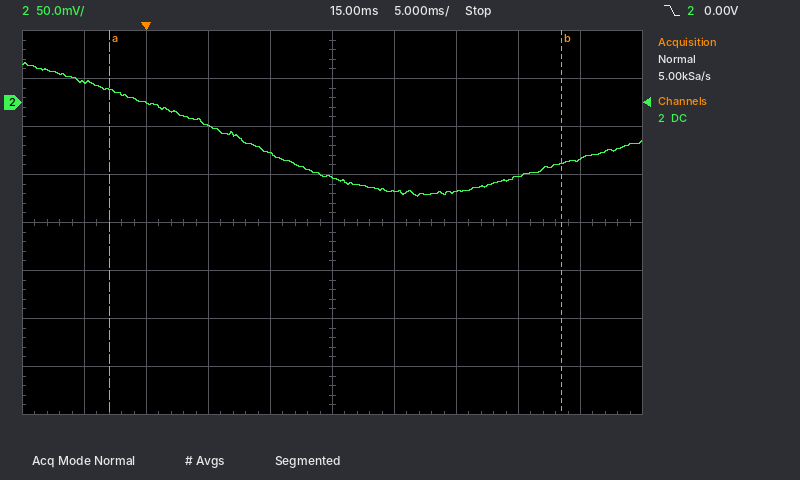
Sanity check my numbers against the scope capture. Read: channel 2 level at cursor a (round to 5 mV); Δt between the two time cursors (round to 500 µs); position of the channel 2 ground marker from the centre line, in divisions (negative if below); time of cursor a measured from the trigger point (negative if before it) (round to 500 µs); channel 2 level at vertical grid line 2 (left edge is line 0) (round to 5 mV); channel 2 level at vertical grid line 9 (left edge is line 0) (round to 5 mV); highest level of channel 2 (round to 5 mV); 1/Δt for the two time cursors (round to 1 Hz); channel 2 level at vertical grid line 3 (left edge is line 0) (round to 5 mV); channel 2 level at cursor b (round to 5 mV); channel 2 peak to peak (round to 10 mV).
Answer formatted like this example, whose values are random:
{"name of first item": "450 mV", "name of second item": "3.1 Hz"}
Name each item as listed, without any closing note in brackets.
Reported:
{"channel 2 level at cursor a": "15 mV", "Δt between the two time cursors": "36.5 ms", "position of the channel 2 ground marker from the centre line, in divisions": "+2.5 div", "time of cursor a measured from the trigger point (negative if before it)": "-3.0 ms", "channel 2 level at vertical grid line 2 (left edge is line 0)": "0 mV", "channel 2 level at vertical grid line 9 (left edge is line 0)": "-60 mV", "highest level of channel 2": "40 mV", "1/Δt for the two time cursors": "27 Hz", "channel 2 level at vertical grid line 3 (left edge is line 0)": "-25 mV", "channel 2 level at cursor b": "-65 mV", "channel 2 peak to peak": "140 mV"}
